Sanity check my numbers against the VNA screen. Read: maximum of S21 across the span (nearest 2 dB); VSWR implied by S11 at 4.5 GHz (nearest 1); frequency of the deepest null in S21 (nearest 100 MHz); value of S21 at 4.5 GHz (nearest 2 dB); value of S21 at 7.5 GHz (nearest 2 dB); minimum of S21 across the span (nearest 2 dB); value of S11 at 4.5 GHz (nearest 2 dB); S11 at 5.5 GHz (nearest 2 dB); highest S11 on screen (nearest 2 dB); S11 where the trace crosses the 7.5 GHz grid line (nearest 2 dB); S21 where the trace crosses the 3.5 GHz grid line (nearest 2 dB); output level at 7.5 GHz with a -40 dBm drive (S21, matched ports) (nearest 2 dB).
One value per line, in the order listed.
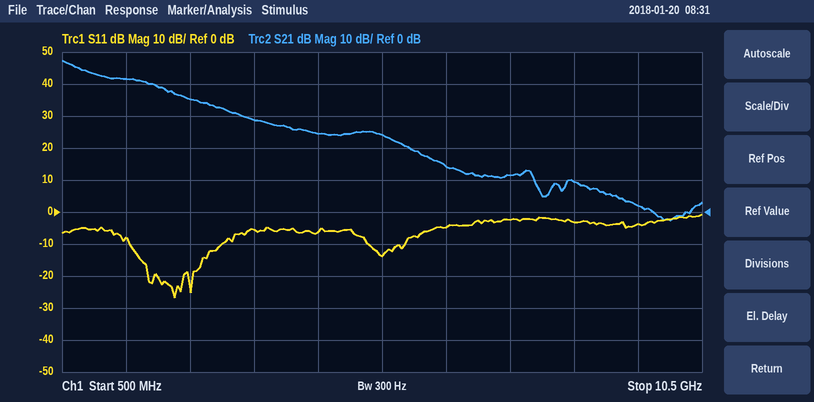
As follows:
48 dB
3
10.0 GHz
24 dB
12 dB
-2 dB
-6 dB
-14 dB
0 dB
-2 dB
28 dB
-28 dBm
